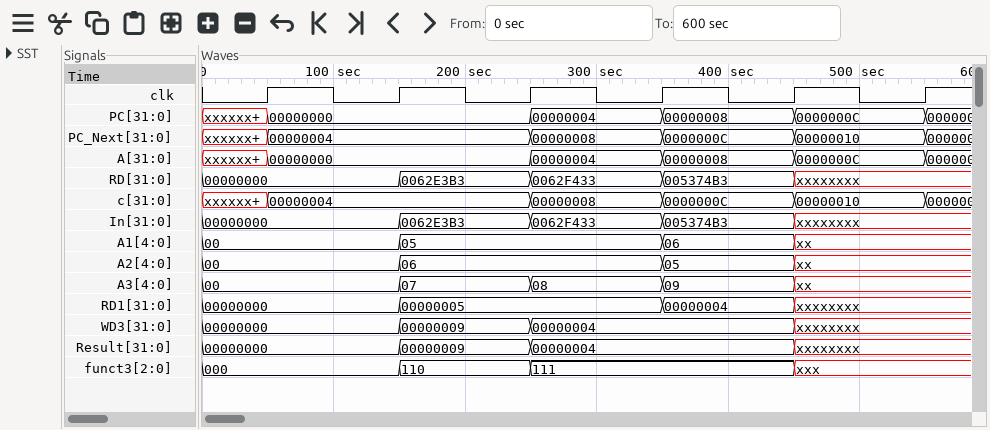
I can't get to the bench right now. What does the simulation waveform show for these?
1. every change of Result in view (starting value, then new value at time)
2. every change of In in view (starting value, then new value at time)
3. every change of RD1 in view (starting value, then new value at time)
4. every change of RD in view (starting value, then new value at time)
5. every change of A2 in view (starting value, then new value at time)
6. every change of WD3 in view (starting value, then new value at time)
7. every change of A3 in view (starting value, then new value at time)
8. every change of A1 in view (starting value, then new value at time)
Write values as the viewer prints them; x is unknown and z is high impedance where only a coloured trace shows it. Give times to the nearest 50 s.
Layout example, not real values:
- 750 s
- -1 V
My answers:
- 00000000, 00000009 at 150 s, 00000004 at 250 s, xxxxxxxx at 450 s
- 00000000, 0062E3B3 at 150 s, 0062F433 at 250 s, 005374B3 at 350 s, xxxxxxxx at 450 s
- 00000000, 00000005 at 150 s, 00000004 at 350 s, xxxxxxxx at 450 s
- 00000000, 0062E3B3 at 150 s, 0062F433 at 250 s, 005374B3 at 350 s, xxxxxxxx at 450 s
- 00, 06 at 150 s, 05 at 350 s, xx at 450 s
- 00000000, 00000009 at 150 s, 00000004 at 250 s, xxxxxxxx at 450 s
- 00, 07 at 150 s, 08 at 250 s, 09 at 350 s, xx at 450 s
- 00, 05 at 150 s, 06 at 350 s, xx at 450 s
